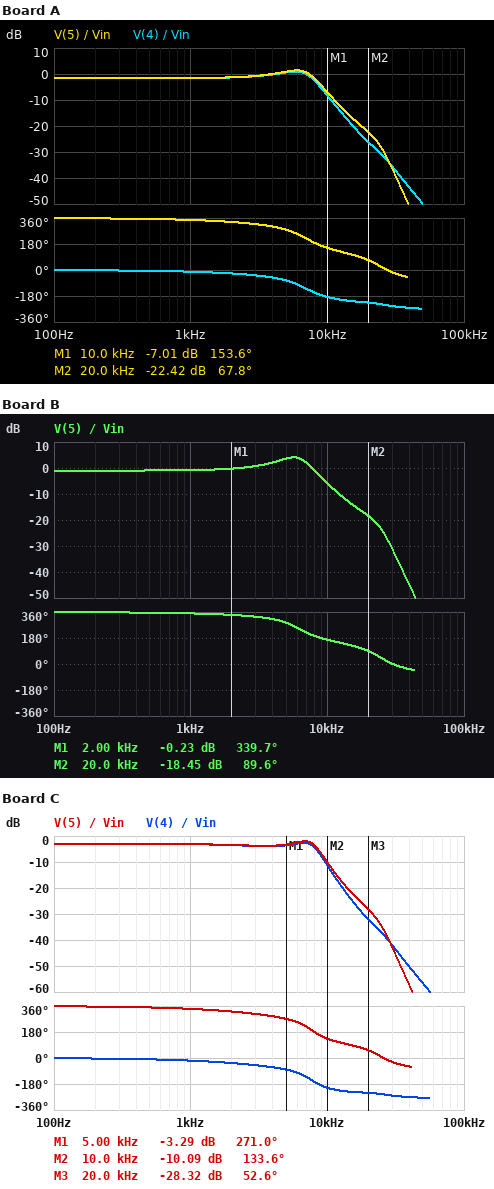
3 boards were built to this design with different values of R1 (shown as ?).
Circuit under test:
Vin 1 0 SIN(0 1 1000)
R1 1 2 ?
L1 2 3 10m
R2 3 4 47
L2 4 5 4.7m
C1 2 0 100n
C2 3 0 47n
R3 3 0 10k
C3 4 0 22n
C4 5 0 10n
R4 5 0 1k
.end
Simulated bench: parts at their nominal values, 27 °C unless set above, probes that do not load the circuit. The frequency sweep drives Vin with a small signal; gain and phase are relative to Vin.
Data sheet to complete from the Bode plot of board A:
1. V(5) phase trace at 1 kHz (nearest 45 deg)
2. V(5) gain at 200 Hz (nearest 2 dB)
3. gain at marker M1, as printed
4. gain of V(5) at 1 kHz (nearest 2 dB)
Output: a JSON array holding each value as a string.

["360 deg", "-2 dB", "-7.01 dB", "-2 dB"]
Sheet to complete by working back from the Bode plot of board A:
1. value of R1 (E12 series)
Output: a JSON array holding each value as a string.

["150 Ω"]
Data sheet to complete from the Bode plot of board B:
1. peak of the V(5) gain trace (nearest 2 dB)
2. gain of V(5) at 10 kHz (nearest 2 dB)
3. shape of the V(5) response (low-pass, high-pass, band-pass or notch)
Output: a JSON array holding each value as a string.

["4 dB", "-6 dB", "low-pass"]
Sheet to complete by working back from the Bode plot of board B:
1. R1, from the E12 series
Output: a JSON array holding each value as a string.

["68 Ω"]
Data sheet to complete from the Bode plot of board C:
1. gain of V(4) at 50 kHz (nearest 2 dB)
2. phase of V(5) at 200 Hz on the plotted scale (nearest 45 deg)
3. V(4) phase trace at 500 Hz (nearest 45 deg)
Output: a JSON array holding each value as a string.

["-56 dB", "360 deg", "0 deg"]
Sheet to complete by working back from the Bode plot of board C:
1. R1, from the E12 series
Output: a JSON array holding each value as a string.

["330 Ω"]
